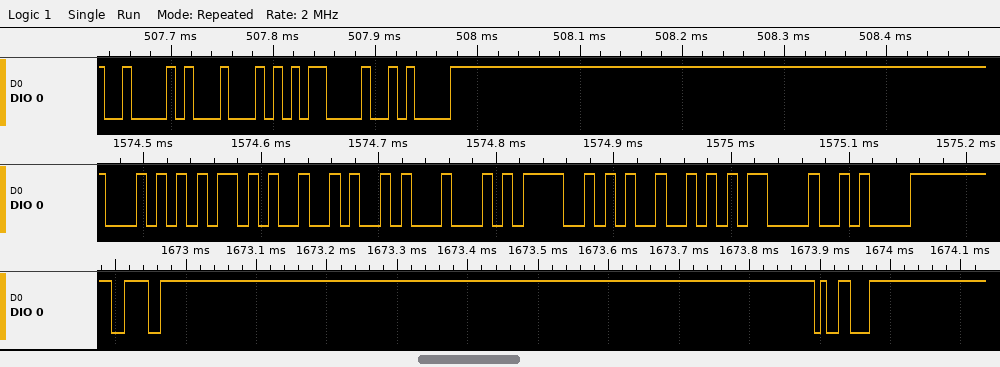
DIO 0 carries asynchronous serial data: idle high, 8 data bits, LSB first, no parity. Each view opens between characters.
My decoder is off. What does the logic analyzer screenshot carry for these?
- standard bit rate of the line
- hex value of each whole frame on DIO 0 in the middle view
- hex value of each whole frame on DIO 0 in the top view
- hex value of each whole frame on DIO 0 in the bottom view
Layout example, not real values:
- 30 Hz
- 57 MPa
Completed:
- 115200 baud
- 54, 2B, 4A, 44, 4F, 49, 0D, 0A
- 42, 44, 0D, 0A
- 9E, 19
